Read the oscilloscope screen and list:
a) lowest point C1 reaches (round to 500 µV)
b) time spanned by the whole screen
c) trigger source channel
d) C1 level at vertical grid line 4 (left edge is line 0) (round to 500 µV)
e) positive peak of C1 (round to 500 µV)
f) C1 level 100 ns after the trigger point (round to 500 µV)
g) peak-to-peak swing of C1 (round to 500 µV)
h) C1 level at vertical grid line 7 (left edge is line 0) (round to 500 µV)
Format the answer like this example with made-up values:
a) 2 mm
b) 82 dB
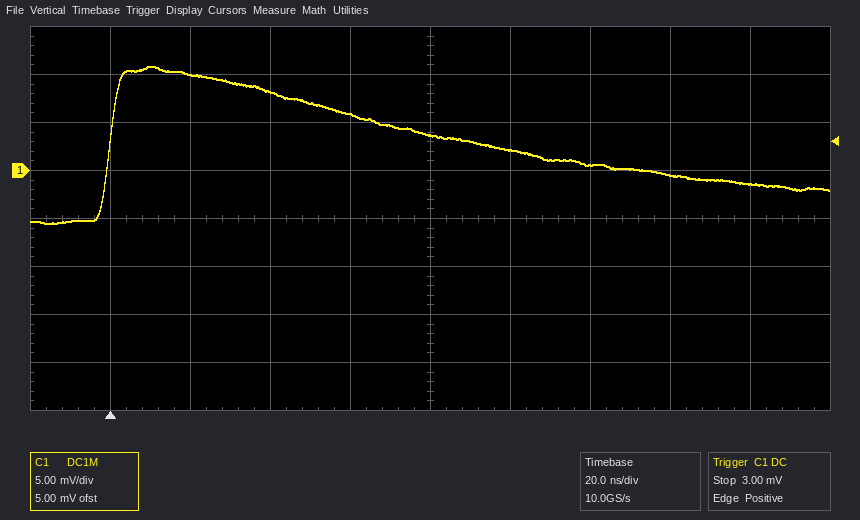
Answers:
a) -5.5 mV
b) 200 ns
c) C1
d) 6.0 mV
e) 11.0 mV
f) 2.0 mV
g) 16.5 mV
h) 500 µV
